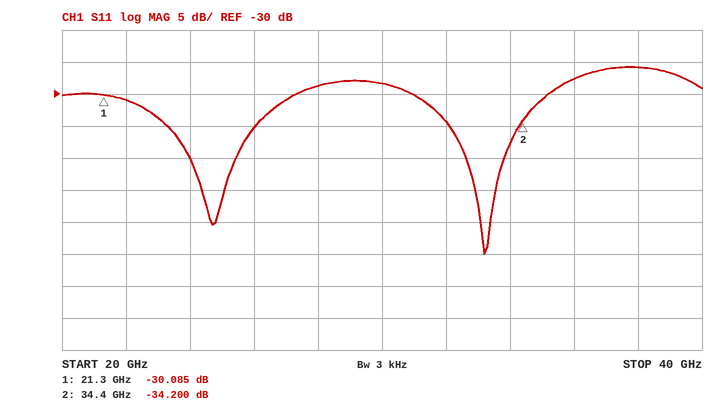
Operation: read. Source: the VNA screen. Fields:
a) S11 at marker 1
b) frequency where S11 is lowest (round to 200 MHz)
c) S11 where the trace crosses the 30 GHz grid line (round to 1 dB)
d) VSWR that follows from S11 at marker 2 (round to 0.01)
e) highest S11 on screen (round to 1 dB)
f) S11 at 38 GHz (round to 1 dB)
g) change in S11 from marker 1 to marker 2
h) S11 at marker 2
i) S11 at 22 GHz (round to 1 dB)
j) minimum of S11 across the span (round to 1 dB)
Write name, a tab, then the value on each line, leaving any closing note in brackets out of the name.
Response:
S11 at marker 1	-30.085 dB
frequency where S11 is lowest	33.2 GHz
S11 where the trace crosses the 30 GHz grid line	-28 dB
VSWR that follows from S11 at marker 2	1.04
highest S11 on screen	-26 dB
S11 at 38 GHz	-26 dB
change in S11 from marker 1 to marker 2	-4.115 dB
S11 at marker 2	-34.200 dB
S11 at 22 GHz	-31 dB
minimum of S11 across the span	-55 dB
